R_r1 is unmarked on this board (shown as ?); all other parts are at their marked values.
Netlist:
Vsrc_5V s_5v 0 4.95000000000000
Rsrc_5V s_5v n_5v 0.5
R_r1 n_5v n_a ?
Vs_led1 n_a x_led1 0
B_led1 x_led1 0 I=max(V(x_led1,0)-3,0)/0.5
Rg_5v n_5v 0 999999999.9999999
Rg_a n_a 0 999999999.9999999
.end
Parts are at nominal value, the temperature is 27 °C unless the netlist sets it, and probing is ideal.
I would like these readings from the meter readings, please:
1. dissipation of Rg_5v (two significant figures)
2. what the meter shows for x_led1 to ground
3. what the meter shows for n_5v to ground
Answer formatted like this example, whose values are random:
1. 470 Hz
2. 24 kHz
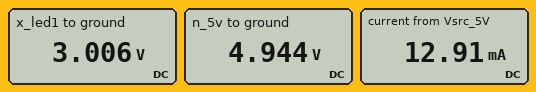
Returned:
1. 24 nW
2. 3.006 V
3. 4.944 V
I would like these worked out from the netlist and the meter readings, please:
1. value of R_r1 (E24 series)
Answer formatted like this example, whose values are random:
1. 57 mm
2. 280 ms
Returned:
1. 150 Ω
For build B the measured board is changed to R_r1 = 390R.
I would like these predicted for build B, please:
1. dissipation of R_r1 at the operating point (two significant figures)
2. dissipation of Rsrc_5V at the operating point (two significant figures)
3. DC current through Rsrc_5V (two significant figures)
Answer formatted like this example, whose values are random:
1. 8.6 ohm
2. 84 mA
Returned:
1. 9.7 mW
2. 12 µW
3. 5.0 mA
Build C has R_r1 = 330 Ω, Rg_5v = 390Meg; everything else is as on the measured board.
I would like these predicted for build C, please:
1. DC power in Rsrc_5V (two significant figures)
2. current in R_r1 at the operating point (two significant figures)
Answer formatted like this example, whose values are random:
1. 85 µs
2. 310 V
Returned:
1. 17 µW
2. 5.9 mA
